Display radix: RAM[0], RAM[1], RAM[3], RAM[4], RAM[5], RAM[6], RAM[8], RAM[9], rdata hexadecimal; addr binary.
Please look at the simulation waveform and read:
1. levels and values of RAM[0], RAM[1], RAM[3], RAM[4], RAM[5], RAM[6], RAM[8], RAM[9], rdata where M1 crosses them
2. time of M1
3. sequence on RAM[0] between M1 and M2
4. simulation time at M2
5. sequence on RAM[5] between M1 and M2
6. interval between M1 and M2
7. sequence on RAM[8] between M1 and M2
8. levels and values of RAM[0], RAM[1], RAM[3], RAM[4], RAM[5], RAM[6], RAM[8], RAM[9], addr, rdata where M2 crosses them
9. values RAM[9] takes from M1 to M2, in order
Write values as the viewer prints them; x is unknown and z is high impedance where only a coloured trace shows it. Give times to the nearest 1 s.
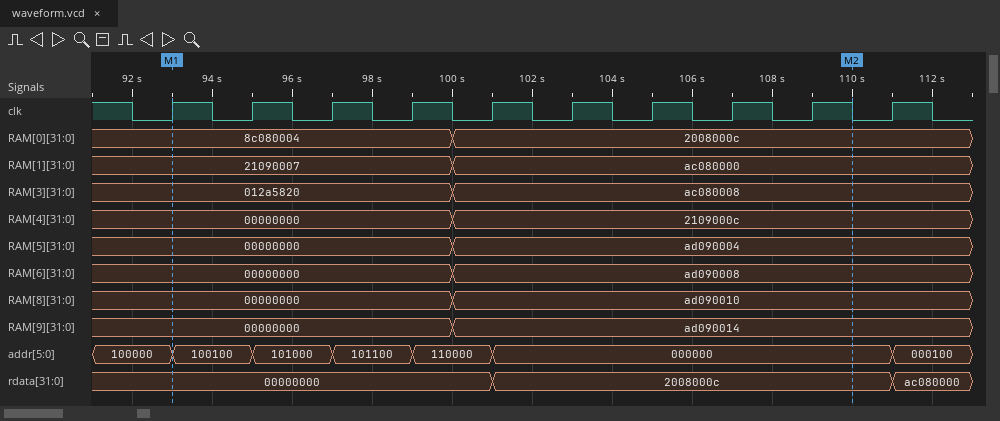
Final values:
RAM[0]=8c080004, RAM[1]=21090007, RAM[3]=012a5820, RAM[4]=00000000, RAM[5]=00000000, RAM[6]=00000000, RAM[8]=00000000, RAM[9]=00000000, rdata=00000000
93 s
8c080004, 2008000c
110 s
00000000, ad090004
17 s
00000000, ad090010
RAM[0]=2008000c, RAM[1]=ac080000, RAM[3]=ac080008, RAM[4]=2109000c, RAM[5]=ad090004, RAM[6]=ad090008, RAM[8]=ad090010, RAM[9]=ad090014, addr=000000, rdata=2008000c
00000000, ad090014
